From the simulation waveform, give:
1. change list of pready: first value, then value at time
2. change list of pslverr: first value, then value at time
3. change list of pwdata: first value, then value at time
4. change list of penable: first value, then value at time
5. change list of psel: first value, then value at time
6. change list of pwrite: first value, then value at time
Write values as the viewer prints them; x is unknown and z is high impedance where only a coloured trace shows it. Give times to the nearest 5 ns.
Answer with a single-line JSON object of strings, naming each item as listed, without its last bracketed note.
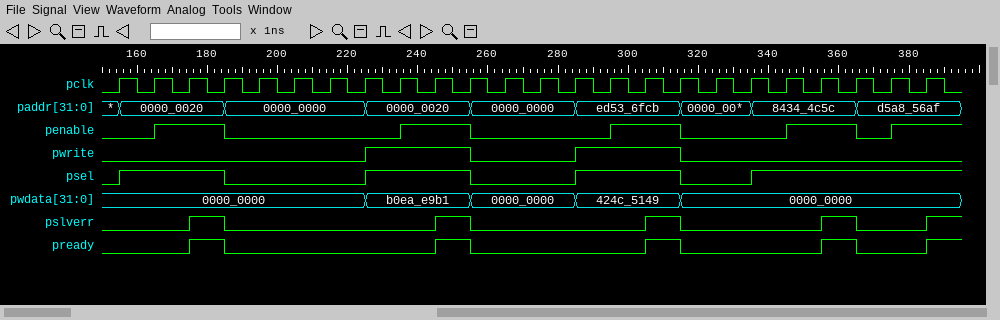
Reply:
{"change list of pready: first value, then value at time": "0, 1 at 175 ns, 0 at 185 ns, 1 at 245 ns, 0 at 255 ns, 1 at 305 ns, 0 at 315 ns, 1 at 355 ns, 0 at 365 ns, 1 at 385 ns", "change list of pslverr: first value, then value at time": "0, 1 at 175 ns, 0 at 185 ns, 1 at 245 ns, 0 at 255 ns, 1 at 305 ns, 0 at 315 ns, 1 at 355 ns, 0 at 365 ns, 1 at 385 ns", "change list of pwdata: first value, then value at time": "0000_0000, b0ea_e9b1 at 225 ns, 0000_0000 at 255 ns, 424c_5149 at 285 ns, 0000_0000 at 315 ns", "change list of penable: first value, then value at time": "0, 1 at 165 ns, 0 at 185 ns, 1 at 235 ns, 0 at 255 ns, 1 at 295 ns, 0 at 315 ns, 1 at 345 ns, 0 at 365 ns, 1 at 375 ns", "change list of psel: first value, then value at time": "0, 1 at 155 ns, 0 at 185 ns, 1 at 225 ns, 0 at 255 ns, 1 at 285 ns, 0 at 315 ns, 1 at 335 ns", "change list of pwrite: first value, then value at time": "0, 1 at 225 ns, 0 at 255 ns, 1 at 285 ns, 0 at 315 ns"}
